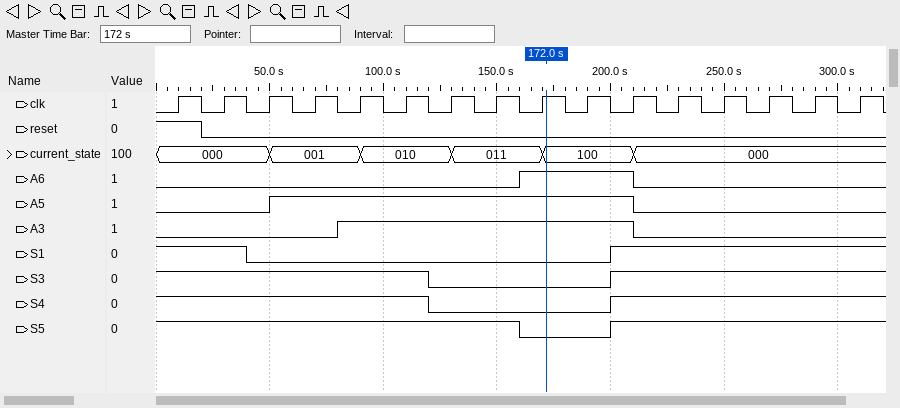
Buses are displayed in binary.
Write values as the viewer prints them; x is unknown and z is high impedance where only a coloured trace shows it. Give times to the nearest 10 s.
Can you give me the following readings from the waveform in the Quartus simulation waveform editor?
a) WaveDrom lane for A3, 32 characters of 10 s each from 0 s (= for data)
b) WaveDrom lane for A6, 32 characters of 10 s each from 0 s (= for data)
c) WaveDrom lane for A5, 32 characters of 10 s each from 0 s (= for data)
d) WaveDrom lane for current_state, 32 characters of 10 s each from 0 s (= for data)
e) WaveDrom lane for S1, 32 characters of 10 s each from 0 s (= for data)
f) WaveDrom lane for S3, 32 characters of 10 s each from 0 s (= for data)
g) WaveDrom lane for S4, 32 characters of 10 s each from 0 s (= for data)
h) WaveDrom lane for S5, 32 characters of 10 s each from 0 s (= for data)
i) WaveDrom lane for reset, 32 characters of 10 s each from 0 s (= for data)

{name: 'A3', wave: '0.......1............0..........'}
{name: 'A6', wave: '0...............1....0..........'}
{name: 'A5', wave: '0....1...............0..........'}
{name: 'current_state', wave: '=....=...=...=...=...=..........', data: '000 001 010 011 100 000'}
{name: 'S1', wave: '1...0...............1...........'}
{name: 'S3', wave: '1...........0.......1...........'}
{name: 'S4', wave: '1...........0.......1...........'}
{name: 'S5', wave: '1...............0...1...........'}
{name: 'reset', wave: '1.0.............................'}
